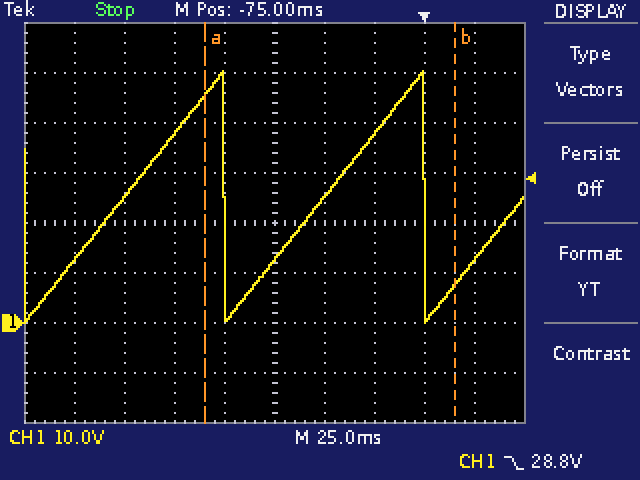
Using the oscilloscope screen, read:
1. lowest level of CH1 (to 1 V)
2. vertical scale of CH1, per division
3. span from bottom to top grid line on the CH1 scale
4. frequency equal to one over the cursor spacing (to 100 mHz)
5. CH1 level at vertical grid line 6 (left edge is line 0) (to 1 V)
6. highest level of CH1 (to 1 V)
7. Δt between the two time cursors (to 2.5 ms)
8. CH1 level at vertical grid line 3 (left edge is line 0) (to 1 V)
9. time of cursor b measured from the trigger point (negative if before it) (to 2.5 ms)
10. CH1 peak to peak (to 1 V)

0 V
10 V
80 V
8.0 Hz
25 V
50 V
125.0 ms
38 V
+15.0 ms
50 V
